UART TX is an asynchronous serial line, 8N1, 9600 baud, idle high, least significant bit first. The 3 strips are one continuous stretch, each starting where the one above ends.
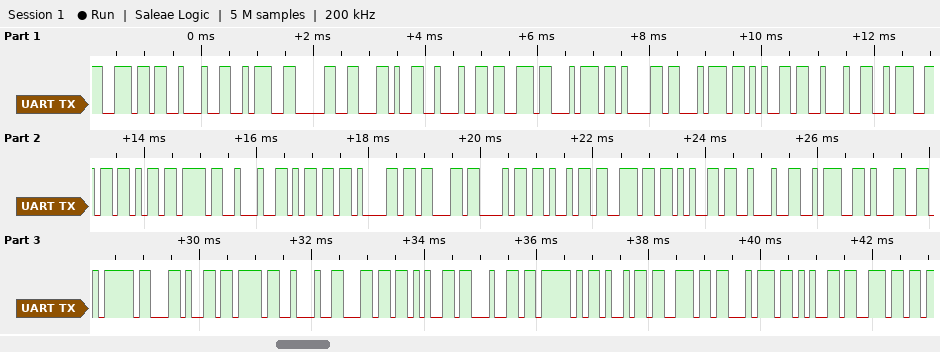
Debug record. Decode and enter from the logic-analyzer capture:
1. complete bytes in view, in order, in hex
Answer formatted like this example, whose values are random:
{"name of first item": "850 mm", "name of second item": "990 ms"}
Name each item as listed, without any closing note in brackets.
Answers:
{"complete bytes in view, in order, in hex": "6E 22 3A 30 2C 22 73 74 61 74 65 22 3A 5B 7B 22 6D 61 63 68 69 6E 65 22 3A 31 7D 2C 7B 22 6C 65 64 5F 69 6E 74 65 6E"}
